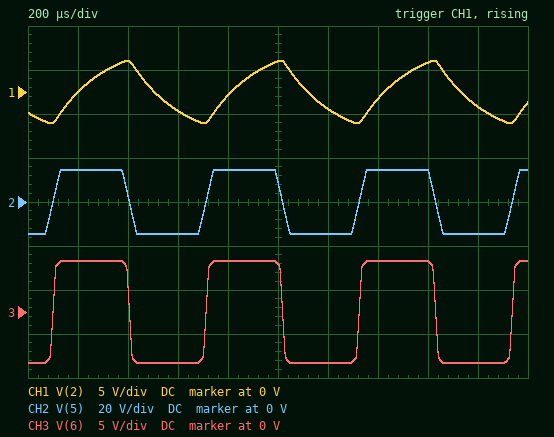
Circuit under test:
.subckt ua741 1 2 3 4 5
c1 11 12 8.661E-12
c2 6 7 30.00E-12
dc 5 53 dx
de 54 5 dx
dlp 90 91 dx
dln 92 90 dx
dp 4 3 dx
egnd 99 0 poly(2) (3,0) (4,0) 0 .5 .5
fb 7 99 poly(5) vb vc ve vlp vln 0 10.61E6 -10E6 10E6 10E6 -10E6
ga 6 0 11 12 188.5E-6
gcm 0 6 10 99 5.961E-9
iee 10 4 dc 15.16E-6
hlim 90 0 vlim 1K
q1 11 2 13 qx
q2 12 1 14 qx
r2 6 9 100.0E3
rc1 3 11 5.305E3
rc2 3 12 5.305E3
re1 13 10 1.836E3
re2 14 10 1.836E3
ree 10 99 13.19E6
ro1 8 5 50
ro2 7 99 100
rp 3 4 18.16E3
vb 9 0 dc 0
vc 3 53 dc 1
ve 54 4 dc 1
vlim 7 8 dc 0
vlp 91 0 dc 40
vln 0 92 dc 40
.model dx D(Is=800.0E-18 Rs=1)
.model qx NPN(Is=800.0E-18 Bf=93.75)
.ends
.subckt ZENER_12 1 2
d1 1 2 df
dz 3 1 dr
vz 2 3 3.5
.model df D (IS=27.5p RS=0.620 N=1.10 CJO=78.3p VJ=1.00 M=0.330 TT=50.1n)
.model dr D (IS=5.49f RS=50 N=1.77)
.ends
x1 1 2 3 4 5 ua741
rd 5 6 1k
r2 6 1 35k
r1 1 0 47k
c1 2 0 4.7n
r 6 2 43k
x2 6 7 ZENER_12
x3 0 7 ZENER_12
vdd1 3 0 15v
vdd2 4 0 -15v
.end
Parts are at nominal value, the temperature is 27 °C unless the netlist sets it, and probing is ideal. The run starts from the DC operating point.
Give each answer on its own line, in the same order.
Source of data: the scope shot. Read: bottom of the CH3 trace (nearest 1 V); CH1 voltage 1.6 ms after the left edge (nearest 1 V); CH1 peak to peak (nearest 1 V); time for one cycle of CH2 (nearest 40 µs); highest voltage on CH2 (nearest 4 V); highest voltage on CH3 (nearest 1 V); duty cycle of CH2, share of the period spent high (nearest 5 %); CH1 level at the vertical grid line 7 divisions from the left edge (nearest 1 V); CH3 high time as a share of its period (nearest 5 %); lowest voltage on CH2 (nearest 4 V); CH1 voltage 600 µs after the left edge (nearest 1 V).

-6 V
3 V
7 V
600 µs
16 V
6 V
50 %
-1 V
50 %
-16 V
-2 V
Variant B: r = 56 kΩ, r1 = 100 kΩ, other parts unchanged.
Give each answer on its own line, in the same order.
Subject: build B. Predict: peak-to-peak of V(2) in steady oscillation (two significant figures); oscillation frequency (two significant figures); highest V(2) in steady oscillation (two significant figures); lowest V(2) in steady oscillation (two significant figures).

8.8 V
920 Hz
4.4 V
-4.4 V
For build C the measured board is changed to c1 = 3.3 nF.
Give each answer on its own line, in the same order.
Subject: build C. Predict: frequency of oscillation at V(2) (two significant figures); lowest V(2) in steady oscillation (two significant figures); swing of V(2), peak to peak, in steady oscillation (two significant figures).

2.2 kHz
-3.7 V
7.3 V
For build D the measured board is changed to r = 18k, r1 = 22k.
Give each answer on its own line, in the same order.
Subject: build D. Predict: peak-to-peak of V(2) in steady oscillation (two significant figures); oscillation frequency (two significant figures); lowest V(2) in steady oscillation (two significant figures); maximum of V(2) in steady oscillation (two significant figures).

6.1 V
4.4 kHz
-3.0 V
3.0 V
